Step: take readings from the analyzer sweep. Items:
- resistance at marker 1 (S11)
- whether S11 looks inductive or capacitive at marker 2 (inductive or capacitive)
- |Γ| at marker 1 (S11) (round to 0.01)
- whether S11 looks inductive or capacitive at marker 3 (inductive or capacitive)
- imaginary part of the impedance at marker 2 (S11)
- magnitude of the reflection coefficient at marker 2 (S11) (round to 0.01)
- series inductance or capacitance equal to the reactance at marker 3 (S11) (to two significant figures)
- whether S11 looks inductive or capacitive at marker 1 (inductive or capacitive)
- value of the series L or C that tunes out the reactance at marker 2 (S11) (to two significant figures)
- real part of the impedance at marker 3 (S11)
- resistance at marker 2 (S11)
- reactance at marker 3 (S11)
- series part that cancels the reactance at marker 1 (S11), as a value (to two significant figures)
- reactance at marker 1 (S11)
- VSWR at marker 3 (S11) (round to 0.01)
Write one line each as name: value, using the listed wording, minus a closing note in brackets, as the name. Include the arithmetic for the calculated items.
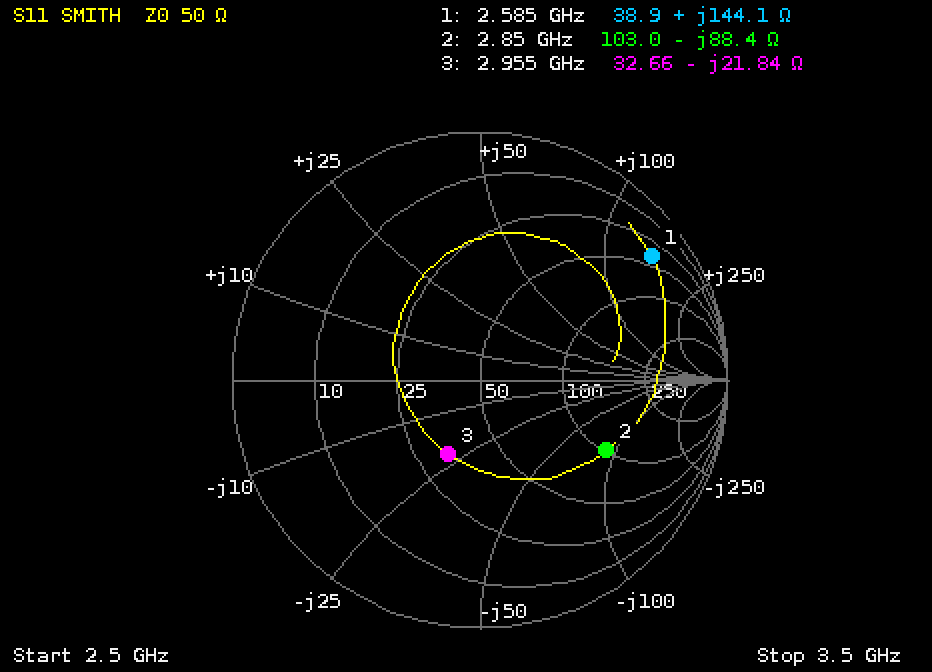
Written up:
resistance at marker 1: 38.9 Ω
whether S11 looks inductive or capacitive at marker 2: capacitive
|Γ| at marker 1 (S11): 0.85
whether S11 looks inductive or capacitive at marker 3: capacitive
imaginary part of the impedance at marker 2: -88.4 Ω
magnitude of the reflection coefficient at marker 2 (S11): 0.58
series inductance or capacitance equal to the reactance at marker 3 (S11): C = 1/(2π × 2.955 GHz × 21.84 Ω) ≈ 2.5 pF
whether S11 looks inductive or capacitive at marker 1: inductive
value of the series L or C that tunes out the reactance at marker 2 (S11): L = 88.4 Ω/(2π × 2.85 GHz) ≈ 4.9 nH
real part of the impedance at marker 3: 32.66 Ω
resistance at marker 2: 103.0 Ω
reactance at marker 3: -21.84 Ω
series part that cancels the reactance at marker 1 (S11), as a value: C = 1/(2π × 2.585 GHz × 144.1 Ω) ≈ 427 fF, so 430 fF to two significant figures
reactance at marker 1: +144.1 Ω
VSWR at marker 3 (S11): 1.97
